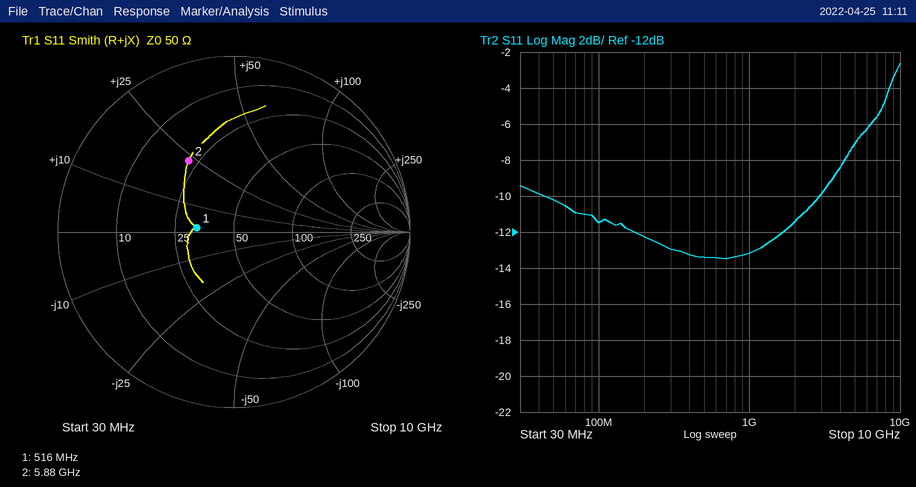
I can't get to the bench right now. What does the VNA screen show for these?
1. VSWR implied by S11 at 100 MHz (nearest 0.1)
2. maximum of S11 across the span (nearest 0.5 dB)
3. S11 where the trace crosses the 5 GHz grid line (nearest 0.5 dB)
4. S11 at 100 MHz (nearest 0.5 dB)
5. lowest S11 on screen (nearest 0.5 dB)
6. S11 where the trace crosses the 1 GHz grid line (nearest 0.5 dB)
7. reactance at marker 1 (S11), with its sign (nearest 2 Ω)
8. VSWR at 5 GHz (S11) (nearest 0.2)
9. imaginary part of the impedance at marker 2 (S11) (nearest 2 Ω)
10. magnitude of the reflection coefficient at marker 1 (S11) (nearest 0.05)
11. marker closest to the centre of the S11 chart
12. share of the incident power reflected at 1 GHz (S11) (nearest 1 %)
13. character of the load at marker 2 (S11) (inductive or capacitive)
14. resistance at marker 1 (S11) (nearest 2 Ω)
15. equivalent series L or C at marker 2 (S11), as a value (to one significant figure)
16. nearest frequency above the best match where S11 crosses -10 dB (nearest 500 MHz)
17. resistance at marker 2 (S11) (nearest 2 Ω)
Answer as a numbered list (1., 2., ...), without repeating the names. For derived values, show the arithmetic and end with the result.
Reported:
1. |Γ| = 10^(-11.5/20) = 0.2661; VSWR = (1 + 0.2661)/(1 − 0.2661) ≈ 1.7
2. -2.5 dB
3. -7.0 dB
4. -11.5 dB
5. -13.5 dB
6. -13.0 dB
7. +2 Ω
8. |Γ| = 10^(-7/20) = 0.4467; VSWR = (1 + 0.4467)/(1 − 0.4467) ≈ 2.6
9. +24 Ω
10. 0.20
11. marker 1
12. 10^(-13/10) ≈ 5 %
13. inductive
14. 32 Ω
15. L = 24 Ω/(2π × 5.88 GHz) ≈ 650 pH, so 600 pH to one significant figure
16. 3.0 GHz
17. 22 Ω
